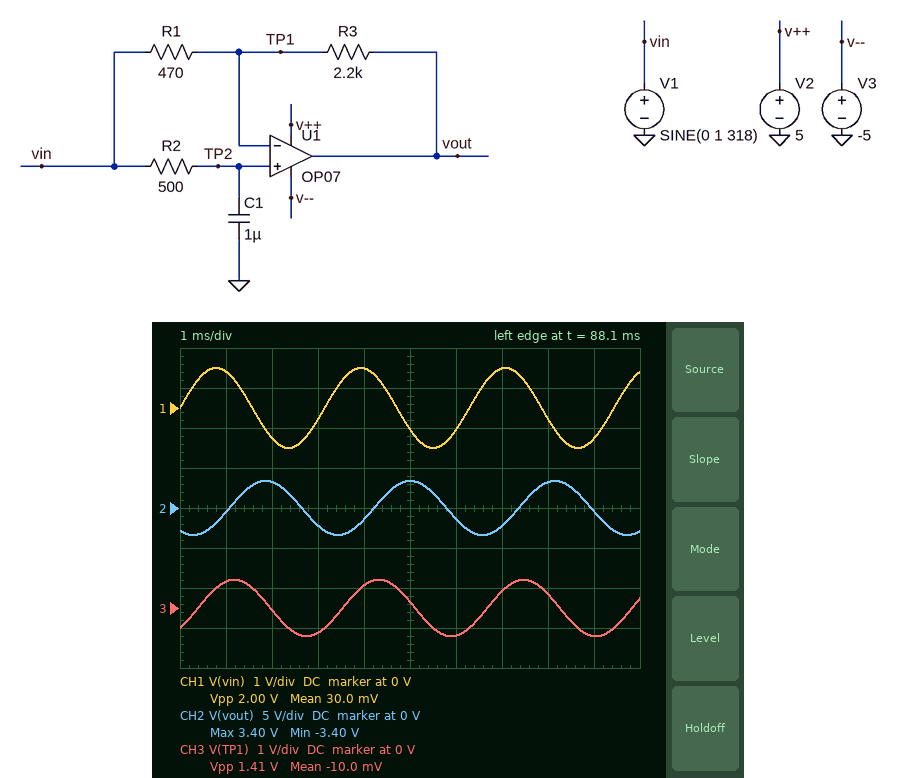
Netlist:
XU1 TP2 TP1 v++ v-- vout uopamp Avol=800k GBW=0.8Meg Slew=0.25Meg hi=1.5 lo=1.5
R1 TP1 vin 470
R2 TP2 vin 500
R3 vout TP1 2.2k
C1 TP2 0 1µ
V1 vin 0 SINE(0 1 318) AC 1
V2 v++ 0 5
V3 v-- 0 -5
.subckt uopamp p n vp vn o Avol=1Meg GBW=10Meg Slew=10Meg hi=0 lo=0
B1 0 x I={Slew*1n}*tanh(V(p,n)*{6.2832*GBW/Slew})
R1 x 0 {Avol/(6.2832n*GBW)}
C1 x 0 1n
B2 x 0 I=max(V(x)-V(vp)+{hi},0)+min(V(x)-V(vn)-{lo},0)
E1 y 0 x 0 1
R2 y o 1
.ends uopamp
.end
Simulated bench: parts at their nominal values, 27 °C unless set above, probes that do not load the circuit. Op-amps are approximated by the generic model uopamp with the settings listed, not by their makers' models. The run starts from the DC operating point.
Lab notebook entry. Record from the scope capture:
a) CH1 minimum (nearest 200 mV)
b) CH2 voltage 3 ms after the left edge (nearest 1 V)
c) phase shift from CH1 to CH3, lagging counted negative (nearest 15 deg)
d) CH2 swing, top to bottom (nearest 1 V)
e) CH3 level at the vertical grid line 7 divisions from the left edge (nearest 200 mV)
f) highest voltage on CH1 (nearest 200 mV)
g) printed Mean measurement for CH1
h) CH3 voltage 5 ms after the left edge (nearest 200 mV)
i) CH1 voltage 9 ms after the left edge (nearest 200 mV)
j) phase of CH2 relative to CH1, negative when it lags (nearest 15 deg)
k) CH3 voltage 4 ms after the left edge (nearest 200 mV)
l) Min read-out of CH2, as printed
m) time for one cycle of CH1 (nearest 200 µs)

-1.0 V
-2 V
-45 deg
7 V
400 mV
1.0 V
30.0 mV
200 mV
-800 mV
-120 deg
600 mV
-3.40 V
3.2 ms
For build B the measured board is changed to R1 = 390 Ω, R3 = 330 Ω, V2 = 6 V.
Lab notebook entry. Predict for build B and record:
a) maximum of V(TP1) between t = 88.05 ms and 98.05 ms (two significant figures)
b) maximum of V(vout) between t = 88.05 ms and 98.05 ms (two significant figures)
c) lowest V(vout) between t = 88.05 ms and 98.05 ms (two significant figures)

710 mV
930 mV
-930 mV
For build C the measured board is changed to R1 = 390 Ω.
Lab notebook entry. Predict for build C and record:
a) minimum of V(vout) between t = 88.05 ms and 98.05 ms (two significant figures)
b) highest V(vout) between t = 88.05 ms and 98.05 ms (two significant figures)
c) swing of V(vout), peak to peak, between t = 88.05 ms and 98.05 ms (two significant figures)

-3.5 V
3.5 V
7.0 V
